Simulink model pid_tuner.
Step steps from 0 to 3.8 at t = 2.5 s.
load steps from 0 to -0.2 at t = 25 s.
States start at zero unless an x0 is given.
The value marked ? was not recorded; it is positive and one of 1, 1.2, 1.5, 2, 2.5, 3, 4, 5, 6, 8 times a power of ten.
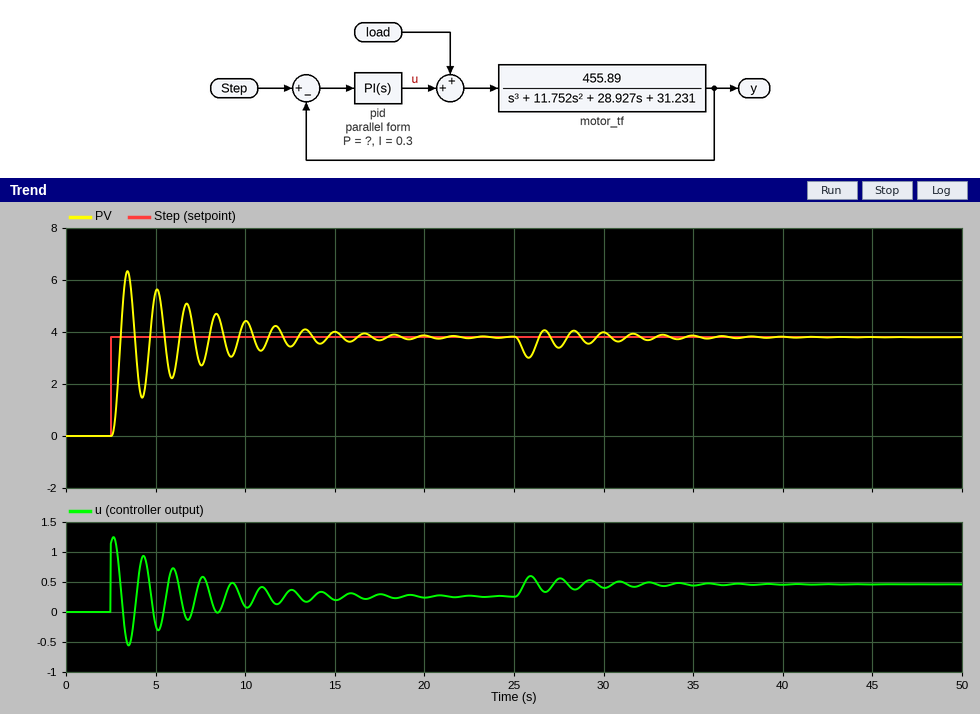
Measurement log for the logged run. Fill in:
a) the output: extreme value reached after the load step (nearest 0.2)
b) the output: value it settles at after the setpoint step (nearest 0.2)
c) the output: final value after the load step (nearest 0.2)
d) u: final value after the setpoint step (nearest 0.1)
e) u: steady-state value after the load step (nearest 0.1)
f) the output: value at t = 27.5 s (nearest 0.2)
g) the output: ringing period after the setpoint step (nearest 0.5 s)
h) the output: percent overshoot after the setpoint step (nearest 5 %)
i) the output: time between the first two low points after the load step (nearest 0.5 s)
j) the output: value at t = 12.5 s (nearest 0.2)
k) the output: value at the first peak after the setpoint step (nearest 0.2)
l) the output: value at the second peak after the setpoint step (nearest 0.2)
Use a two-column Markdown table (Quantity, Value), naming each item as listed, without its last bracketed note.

| Quantity | Value |
|---|---|
| the output: extreme value reached after the load step | 3.0 |
| the output: value it settles at after the setpoint step | 3.8 |
| the output: final value after the load step | 3.8 |
| u: final value after the setpoint step | 0.3 |
| u: steady-state value after the load step | 0.5 |
| the output: value at t = 27.5 s | 3.4 |
| the output: ringing period after the setpoint step | 1.5 s |
| the output: percent overshoot after the setpoint step | 65 % |
| the output: time between the first two low points after the load step | 1.5 s |
| the output: value at t = 12.5 s | 3.4 |
| the output: value at the first peak after the setpoint step | 6.4 |
| the output: value at the second peak after the setpoint step | 5.6 |
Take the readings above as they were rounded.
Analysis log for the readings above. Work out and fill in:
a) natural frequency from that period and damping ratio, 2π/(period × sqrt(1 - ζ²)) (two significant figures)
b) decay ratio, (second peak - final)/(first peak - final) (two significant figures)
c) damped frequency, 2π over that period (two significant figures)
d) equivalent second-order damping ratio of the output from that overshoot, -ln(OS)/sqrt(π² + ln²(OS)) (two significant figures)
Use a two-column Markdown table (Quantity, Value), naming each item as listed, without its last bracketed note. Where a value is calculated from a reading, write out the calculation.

| Quantity | Value |
|---|---|
| natural frequency from that period and damping ratio, 2π/(period × sqrt(1 - ζ²)) | 2π / (1.5 × sqrt(1 - 0.14²)) = 4.2 rad/s |
| decay ratio, (second peak - final)/(first peak - final) | (5.6 - 3.8) / (6.4 - 3.8) = 0.69 |
| damped frequency, 2π over that period | 2π / 1.5 = 4.2 rad/s |
| equivalent second-order damping ratio of the output from that overshoot, -ln(OS)/sqrt(π² + ln²(OS)) | ln(0.65) = -0.431; 0.431 / sqrt(9.870 + 0.186) = 0.14 |
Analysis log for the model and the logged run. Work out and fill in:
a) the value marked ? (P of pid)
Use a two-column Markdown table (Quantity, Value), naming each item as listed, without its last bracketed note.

| Quantity | Value |
|---|---|
| the value marked ? | 0.3 |
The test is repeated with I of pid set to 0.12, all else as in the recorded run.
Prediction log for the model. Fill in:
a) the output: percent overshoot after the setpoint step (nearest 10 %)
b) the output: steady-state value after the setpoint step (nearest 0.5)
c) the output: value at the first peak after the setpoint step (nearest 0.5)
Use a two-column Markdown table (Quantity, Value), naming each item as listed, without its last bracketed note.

| Quantity | Value |
|---|---|
| the output: percent overshoot after the setpoint step | 40 % |
| the output: steady-state value after the setpoint step | 4.0 |
| the output: value at the first peak after the setpoint step | 5.5 |
